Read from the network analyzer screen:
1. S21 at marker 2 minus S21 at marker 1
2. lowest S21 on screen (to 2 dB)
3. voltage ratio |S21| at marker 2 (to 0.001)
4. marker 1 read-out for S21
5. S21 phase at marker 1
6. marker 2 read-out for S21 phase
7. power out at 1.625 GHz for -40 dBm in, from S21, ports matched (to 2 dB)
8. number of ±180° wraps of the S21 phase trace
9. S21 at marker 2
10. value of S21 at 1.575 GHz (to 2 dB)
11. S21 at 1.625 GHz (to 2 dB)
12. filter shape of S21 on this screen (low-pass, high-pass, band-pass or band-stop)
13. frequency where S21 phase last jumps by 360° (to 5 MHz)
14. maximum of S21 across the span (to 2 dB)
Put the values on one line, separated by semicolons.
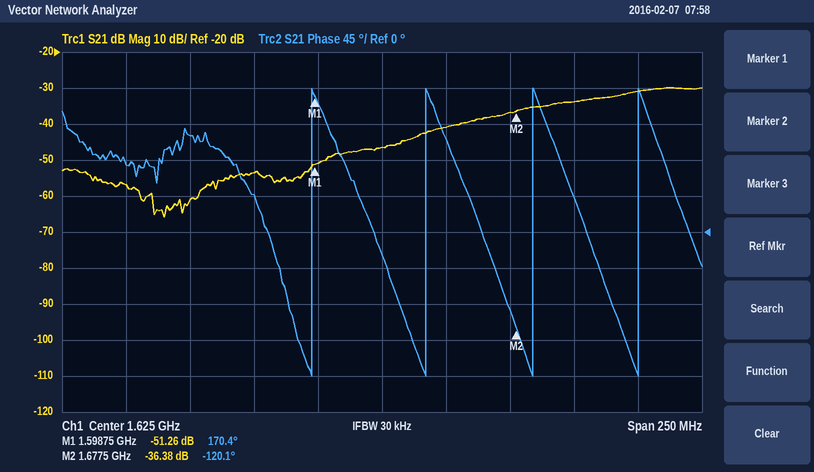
14.88 dB; -66 dB; 0.015; -51.26 dB; 170.4°; -120.1°; -86 dBm; 4; -36.38 dB; -54 dB; -46 dB; high-pass; 1.725 GHz; -30 dB
